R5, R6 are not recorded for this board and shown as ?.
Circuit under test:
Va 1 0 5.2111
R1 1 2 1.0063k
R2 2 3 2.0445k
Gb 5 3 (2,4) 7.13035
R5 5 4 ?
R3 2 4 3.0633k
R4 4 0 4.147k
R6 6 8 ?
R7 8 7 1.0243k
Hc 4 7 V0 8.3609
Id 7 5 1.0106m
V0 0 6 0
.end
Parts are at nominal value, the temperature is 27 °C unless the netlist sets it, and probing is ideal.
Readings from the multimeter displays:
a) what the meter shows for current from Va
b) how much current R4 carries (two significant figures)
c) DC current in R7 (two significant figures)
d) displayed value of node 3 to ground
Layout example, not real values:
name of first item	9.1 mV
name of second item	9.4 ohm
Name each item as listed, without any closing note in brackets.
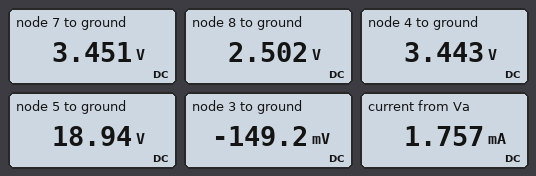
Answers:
what the meter shows for current from Va	1.757 mA
how much current R4 carries	830 µA
DC current in R7	930 µA
displayed value of node 3 to ground	-149.2 mV
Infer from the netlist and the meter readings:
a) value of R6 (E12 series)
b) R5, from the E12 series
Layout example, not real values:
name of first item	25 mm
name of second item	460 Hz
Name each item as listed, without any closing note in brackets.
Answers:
value of R6	2.7 kΩ
R5, from the E12 series	5.6 kΩ
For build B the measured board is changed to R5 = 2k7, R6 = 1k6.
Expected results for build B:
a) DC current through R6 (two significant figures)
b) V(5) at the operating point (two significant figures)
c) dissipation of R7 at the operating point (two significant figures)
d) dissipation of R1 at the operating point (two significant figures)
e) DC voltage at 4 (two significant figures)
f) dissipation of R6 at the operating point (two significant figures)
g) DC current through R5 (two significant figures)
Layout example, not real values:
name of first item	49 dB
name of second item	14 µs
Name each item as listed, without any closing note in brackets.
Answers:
DC current through R6	1.2 mA
V(5) at the operating point	11 V
dissipation of R7 at the operating point	1.5 mW
dissipation of R1 at the operating point	4.0 mW
DC voltage at 4	3.2 V
dissipation of R6 at the operating point	2.4 mW
DC current through R5	3.0 mA
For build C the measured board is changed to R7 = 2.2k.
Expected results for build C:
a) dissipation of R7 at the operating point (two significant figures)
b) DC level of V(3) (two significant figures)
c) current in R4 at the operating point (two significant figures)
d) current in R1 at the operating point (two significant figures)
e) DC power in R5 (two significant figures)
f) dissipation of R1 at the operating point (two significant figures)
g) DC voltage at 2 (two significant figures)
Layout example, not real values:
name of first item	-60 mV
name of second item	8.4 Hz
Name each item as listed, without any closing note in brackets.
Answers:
dissipation of R7 at the operating point	1.2 mW
DC level of V(3)	320 mV
current in R4 at the operating point	870 µA
current in R1 at the operating point	1.6 mA
DC power in R5	38 mW
dissipation of R1 at the operating point	2.6 mW
DC voltage at 2	3.6 V
